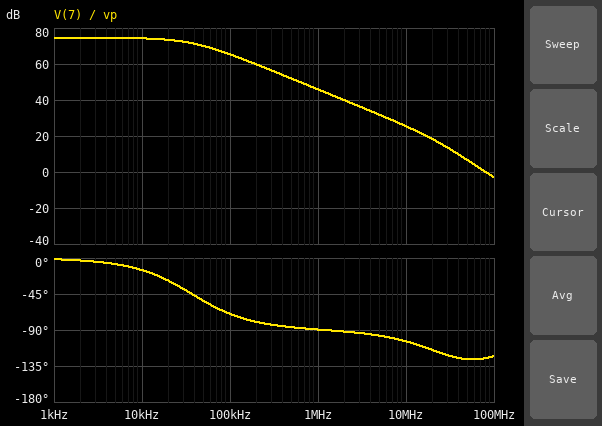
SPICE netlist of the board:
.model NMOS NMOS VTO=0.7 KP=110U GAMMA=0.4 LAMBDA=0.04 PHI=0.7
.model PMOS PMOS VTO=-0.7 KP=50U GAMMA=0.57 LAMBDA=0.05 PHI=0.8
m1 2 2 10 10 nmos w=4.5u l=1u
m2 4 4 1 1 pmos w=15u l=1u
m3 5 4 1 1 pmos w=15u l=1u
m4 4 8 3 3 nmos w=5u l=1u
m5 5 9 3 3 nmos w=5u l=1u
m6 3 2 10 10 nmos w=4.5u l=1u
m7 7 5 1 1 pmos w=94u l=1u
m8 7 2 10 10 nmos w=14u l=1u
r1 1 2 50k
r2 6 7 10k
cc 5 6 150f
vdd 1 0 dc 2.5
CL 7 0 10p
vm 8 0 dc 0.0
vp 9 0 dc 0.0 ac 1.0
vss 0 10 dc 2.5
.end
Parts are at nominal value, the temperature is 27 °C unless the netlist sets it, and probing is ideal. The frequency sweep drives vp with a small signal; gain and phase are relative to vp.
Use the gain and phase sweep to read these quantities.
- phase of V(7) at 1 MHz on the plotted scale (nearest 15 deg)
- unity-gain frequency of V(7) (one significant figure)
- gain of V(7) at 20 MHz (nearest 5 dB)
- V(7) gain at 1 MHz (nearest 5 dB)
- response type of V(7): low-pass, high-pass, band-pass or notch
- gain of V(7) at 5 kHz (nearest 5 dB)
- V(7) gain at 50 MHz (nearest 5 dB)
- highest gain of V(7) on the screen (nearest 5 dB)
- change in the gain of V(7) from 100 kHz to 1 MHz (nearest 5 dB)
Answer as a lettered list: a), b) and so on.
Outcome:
a) -90 deg
b) 80 MHz
c) 20 dB
d) 45 dB
e) low-pass
f) 75 dB
g) 5 dB
h) 75 dB
i) -20 dB
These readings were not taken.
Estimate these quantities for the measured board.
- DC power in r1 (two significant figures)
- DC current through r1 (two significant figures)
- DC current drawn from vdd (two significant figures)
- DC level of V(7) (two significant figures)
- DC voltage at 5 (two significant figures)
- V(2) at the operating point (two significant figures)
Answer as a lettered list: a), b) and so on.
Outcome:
a) 280 µW
b) 75 µA
c) 400 µA
d) 450 mV
e) 1.5 V
f) -1.3 V
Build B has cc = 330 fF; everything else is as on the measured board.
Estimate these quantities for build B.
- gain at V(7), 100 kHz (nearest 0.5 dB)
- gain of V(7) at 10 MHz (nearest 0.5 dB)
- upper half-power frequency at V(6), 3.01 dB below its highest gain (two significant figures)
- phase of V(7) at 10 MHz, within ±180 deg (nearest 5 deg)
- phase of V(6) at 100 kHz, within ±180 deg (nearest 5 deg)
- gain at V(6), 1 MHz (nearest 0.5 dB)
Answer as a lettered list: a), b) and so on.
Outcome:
a) 59.5 dB
b) 19.0 dB
c) 18 kHz
d) -100 deg
e) -80 deg
f) 39.5 dB
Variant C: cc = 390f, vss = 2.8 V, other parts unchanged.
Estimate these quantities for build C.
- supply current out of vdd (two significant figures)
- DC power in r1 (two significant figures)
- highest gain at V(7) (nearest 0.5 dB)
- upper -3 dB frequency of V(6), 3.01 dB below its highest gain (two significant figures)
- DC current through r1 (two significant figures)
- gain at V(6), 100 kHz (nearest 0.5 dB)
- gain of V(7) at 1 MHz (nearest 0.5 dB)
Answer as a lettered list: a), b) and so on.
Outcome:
a) 430 µA
b) 330 µW
c) 74.0 dB
d) 17 kHz
e) 81 µA
f) 58.5 dB
g) 38.5 dB
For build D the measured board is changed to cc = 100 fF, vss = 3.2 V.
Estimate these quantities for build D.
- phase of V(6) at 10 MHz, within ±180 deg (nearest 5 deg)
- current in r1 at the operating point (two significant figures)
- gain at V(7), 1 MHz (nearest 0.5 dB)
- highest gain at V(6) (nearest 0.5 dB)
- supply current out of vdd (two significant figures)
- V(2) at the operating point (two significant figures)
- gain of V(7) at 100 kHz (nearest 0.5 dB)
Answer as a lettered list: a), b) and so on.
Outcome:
a) -105 deg
b) 88 µA
c) 49.5 dB
d) 73.0 dB
e) 480 µA
f) -1.9 V
g) 68.0 dB
